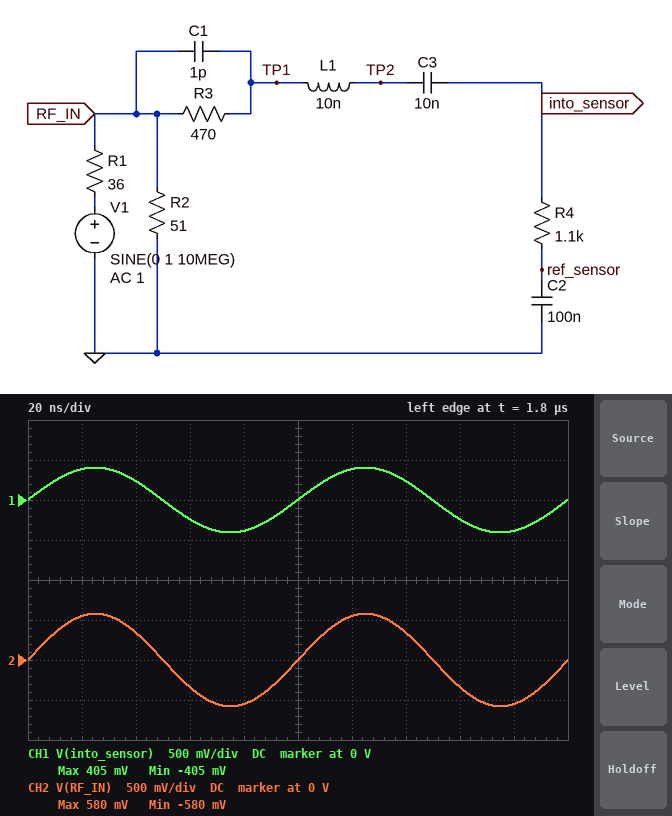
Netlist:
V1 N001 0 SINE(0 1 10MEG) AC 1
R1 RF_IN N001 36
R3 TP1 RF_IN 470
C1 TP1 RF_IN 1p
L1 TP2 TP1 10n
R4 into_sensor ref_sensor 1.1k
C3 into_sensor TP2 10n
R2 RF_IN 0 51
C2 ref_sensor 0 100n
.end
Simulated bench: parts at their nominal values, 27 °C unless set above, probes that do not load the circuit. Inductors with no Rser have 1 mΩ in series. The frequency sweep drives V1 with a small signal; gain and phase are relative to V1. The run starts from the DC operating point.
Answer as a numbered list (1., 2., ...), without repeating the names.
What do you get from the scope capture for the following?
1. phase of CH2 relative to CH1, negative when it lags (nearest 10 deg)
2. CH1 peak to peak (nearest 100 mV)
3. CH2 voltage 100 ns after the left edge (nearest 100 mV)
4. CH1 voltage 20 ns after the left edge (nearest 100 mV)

1. 0 deg
2. 800 mV
3. 0 V
4. 400 mV
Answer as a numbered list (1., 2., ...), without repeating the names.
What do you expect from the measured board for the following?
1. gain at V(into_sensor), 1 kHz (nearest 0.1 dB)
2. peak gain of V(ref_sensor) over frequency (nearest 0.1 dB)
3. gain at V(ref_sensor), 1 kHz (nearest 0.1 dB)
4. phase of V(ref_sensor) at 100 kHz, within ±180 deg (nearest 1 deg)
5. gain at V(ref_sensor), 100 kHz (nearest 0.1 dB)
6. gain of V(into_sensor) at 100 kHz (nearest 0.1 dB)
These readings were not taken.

1. -23.8 dB
2. -25.5 dB
3. -25.5 dB
4. -84 deg
5. -44.7 dB
6. -7.9 dB
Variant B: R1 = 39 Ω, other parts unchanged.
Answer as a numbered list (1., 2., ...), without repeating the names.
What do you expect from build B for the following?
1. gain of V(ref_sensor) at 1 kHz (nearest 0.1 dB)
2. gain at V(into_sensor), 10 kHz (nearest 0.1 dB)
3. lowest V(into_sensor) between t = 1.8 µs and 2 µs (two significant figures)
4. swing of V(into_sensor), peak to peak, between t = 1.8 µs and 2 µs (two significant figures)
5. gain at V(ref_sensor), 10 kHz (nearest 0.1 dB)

1. -25.8 dB
2. -11.5 dB
3. -390 mV
4. 780 mV
5. -28.4 dB
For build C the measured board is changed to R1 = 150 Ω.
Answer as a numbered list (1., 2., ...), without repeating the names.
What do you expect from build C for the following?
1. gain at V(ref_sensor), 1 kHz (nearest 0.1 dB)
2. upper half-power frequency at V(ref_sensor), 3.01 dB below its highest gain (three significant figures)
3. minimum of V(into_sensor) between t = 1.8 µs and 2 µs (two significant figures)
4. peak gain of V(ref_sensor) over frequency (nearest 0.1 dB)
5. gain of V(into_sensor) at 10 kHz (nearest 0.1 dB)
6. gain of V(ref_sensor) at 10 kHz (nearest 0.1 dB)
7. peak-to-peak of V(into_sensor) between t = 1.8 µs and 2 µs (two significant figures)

1. -32.8 dB
2. 10.9 kHz
3. -170 mV
4. -32.7 dB
5. -18.5 dB
6. -35.4 dB
7. 350 mV
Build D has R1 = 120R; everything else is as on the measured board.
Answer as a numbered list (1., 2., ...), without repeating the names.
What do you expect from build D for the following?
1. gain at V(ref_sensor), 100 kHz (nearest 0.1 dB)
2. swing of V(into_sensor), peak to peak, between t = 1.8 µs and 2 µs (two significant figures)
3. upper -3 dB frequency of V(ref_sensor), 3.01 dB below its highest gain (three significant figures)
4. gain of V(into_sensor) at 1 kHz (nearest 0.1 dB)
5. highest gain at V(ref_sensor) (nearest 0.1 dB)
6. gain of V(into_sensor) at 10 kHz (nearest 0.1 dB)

1. -50.6 dB
2. 410 mV
3. 10.9 kHz
4. -29.7 dB
5. -31.3 dB
6. -17.1 dB
